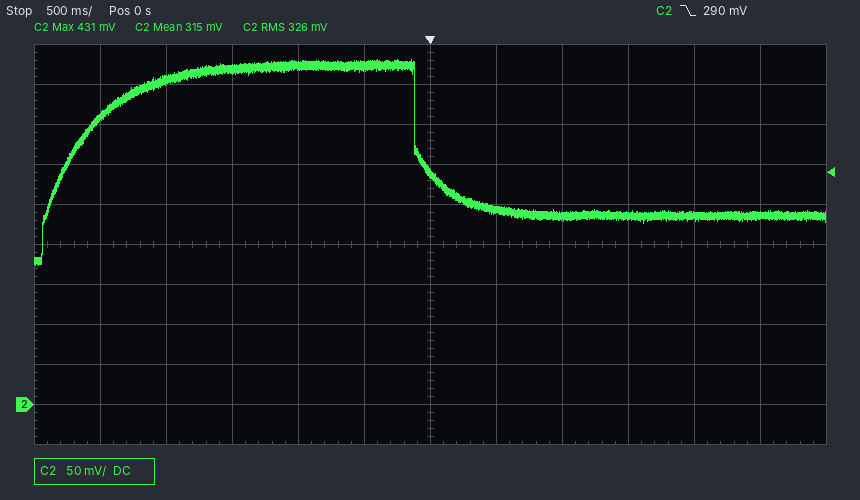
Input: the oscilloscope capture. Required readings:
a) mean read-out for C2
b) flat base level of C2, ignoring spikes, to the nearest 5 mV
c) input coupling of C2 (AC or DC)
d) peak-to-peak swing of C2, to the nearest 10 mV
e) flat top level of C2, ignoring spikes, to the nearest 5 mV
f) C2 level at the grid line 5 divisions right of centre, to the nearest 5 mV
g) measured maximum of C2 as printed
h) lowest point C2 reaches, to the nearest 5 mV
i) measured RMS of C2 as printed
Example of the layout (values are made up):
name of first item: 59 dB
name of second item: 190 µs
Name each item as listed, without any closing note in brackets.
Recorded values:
mean read-out for C2: 315 mV
flat base level of C2, ignoring spikes, to the nearest 5 mV: 235 mV
input coupling of C2: DC
peak-to-peak swing of C2, to the nearest 10 mV: 260 mV
flat top level of C2, ignoring spikes, to the nearest 5 mV: 425 mV
C2 level at the grid line 5 divisions right of centre, to the nearest 5 mV: 235 mV
measured maximum of C2 as printed: 431 mV
lowest point C2 reaches, to the nearest 5 mV: 175 mV
measured RMS of C2 as printed: 326 mV
